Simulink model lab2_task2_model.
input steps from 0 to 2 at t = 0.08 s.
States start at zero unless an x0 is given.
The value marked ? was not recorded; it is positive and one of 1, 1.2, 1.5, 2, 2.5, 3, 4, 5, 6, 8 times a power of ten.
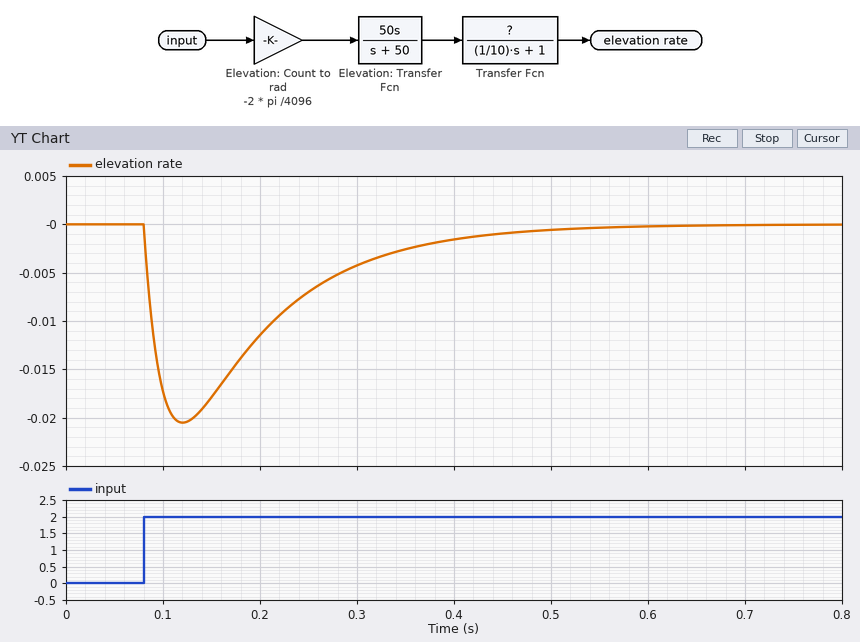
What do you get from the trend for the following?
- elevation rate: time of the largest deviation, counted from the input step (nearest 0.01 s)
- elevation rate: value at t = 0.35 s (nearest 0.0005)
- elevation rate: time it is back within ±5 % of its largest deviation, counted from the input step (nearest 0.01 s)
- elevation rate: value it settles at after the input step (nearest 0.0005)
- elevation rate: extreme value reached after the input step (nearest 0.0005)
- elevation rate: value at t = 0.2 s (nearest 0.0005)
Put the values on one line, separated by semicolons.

0.04 s; -0.0025; 0.36 s; 0.0000; -0.0205; -0.0115
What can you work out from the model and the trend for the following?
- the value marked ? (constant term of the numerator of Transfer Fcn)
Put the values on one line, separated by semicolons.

1
